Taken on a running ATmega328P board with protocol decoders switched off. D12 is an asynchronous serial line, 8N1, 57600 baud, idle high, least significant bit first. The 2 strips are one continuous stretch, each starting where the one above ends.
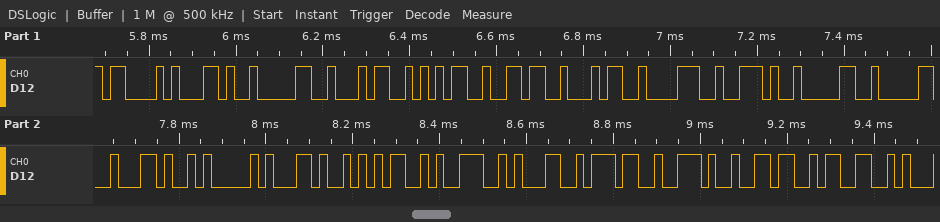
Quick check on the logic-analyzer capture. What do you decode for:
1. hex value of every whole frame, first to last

0x43 0x2C 0x30 0x34 0x35 0x36 0x34 0x38 0x2E 0x30 0x30 0x2C 0x41 0x2C 0x35 0x39 0x31 0x37 0x2E 0x36 0x33
